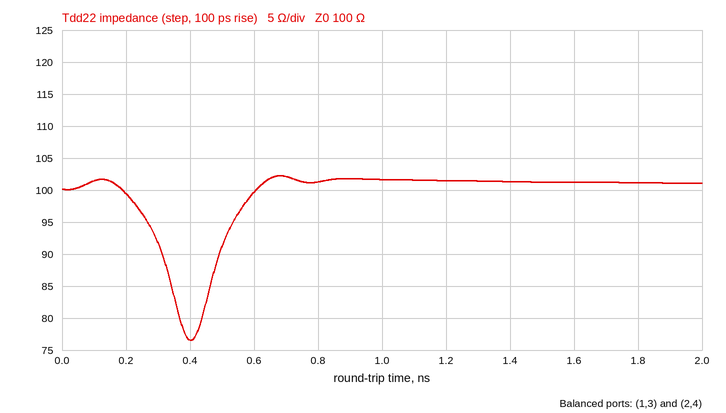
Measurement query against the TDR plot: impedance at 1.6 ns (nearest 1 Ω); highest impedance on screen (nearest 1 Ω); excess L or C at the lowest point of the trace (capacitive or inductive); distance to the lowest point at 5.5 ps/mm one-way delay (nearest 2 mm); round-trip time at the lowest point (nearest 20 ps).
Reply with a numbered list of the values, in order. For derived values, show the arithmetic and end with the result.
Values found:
1. 101 Ω
2. 102 Ω
3. capacitive
4. 400 ps / 2 / 5.5 ps/mm ≈ 36 mm
5. 400 ps
